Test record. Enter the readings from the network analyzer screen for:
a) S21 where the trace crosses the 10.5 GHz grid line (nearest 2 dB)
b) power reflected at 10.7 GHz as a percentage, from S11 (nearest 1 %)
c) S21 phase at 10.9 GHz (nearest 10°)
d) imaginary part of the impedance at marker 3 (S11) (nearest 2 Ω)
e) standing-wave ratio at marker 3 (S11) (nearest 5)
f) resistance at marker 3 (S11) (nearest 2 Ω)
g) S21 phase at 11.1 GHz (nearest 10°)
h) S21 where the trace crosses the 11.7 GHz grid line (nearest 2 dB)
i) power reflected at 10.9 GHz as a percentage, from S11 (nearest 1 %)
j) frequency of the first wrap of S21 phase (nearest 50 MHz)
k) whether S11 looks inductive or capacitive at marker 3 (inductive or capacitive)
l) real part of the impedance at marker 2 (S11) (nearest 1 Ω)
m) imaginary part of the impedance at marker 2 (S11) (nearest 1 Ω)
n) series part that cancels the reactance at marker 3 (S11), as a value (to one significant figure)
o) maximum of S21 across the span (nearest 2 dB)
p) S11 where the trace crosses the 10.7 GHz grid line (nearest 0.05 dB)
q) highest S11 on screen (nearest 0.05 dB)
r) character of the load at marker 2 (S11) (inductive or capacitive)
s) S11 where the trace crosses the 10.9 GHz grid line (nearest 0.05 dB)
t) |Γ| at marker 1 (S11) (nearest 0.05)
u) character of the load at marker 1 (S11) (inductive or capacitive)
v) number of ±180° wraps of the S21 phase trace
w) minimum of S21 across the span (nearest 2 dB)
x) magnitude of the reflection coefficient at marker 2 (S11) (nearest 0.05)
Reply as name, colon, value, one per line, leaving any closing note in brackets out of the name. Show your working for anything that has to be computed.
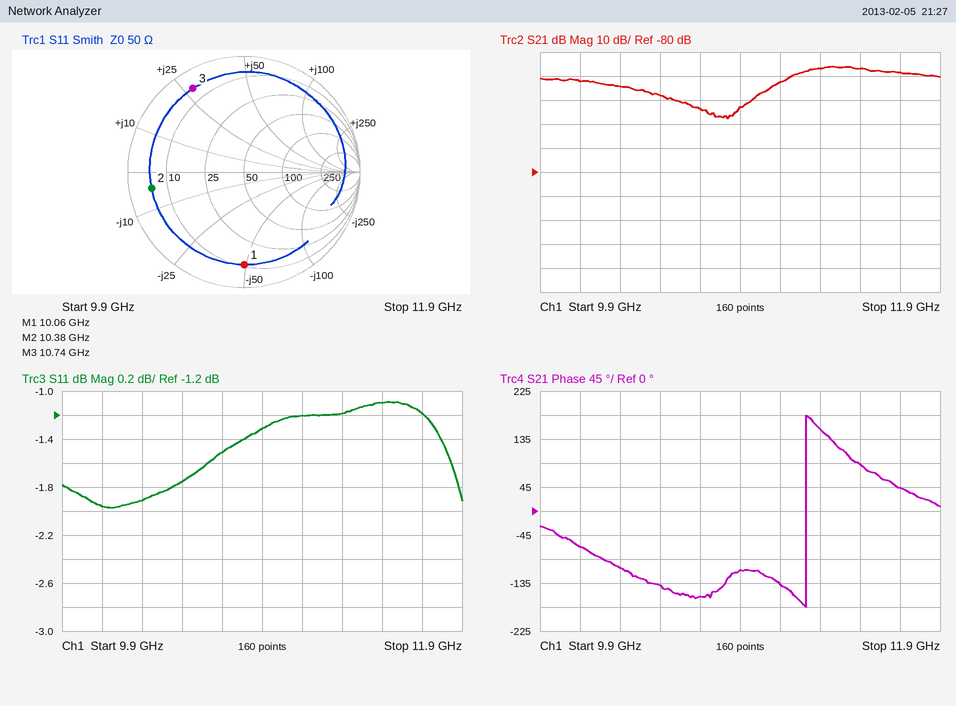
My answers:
S21 where the trace crosses the 10.5 GHz grid line: -48 dB
power reflected at 10.7 GHz as a percentage, from S11: 10^(-1.5/10) ≈ 71 %
S21 phase at 10.9 GHz: -110°
imaginary part of the impedance at marker 3 (S11): +28 Ω
standing-wave ratio at marker 3 (S11): 10
resistance at marker 3 (S11): 6 Ω
S21 phase at 11.1 GHz: -140°
S21 where the trace crosses the 11.7 GHz grid line: -38 dB
power reflected at 10.9 GHz as a percentage, from S11: 10^(-1.3/10) ≈ 74 %
frequency of the first wrap of S21 phase: 11.25 GHz
whether S11 looks inductive or capacitive at marker 3: inductive
real part of the impedance at marker 2 (S11): 5 Ω
imaginary part of the impedance at marker 2 (S11): -4 Ω
series part that cancels the reactance at marker 3 (S11), as a value: C = 1/(2π × 10.74 GHz × 28 Ω) ≈ 529 fF, so 500 fF to one significant figure
maximum of S21 across the span: -36 dB
S11 where the trace crosses the 10.7 GHz grid line: -1.50 dB
highest S11 on screen: -1.10 dB
character of the load at marker 2 (S11): capacitive
S11 where the trace crosses the 10.9 GHz grid line: -1.30 dB
|Γ| at marker 1 (S11): 0.80
character of the load at marker 1 (S11): capacitive
number of ±180° wraps of the S21 phase trace: 1
minimum of S21 across the span: -58 dB
magnitude of the reflection coefficient at marker 2 (S11): 0.80
